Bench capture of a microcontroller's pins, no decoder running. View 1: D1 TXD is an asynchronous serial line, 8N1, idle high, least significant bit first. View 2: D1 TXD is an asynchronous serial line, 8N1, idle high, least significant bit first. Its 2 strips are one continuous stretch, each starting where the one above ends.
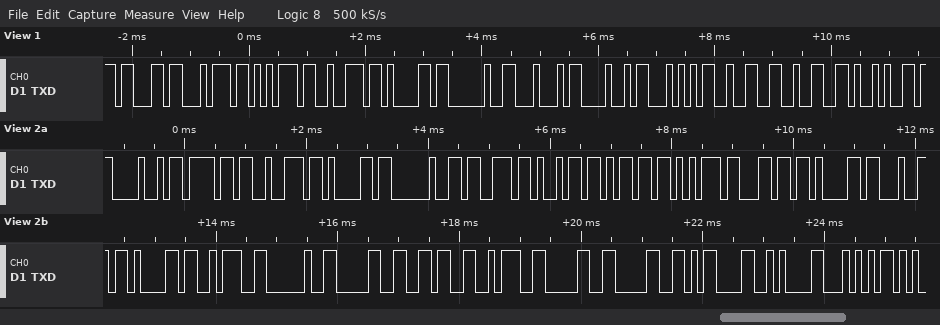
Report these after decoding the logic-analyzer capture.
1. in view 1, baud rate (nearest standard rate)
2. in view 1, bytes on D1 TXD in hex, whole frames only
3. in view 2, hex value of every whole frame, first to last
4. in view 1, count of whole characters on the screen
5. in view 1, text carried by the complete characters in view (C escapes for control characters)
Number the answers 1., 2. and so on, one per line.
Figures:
1. 9600 baud
2. 0x63 0x74 0x75 0x72 0x61 0x20 0x44 0x48 0x54 0x32 0x32 0x29
3. 48 6F 72 61 20 73 69 6D 75 6C 61 64 61 3A 20 30 36 3A 30 30 0D 0A 54
4. 12
5. "ctura DHT22)"
